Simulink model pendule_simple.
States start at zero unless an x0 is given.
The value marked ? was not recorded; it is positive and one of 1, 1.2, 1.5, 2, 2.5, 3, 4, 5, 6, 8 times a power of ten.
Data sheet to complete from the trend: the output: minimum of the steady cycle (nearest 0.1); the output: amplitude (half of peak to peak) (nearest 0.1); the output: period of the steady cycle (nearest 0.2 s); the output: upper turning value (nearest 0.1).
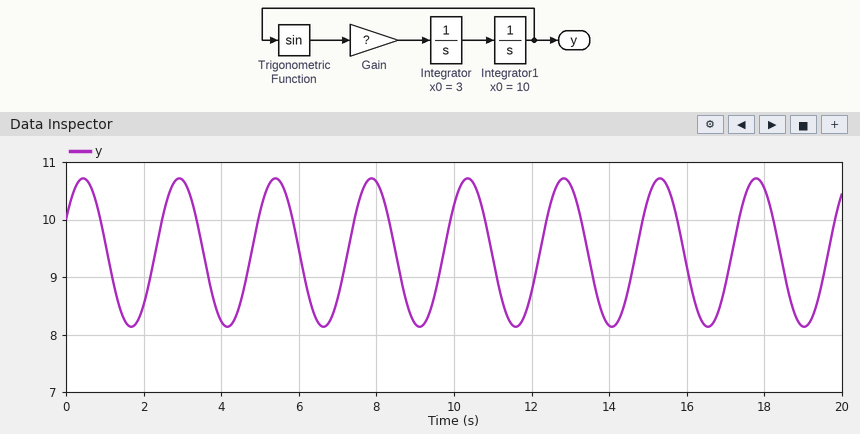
8.1
1.3
2.4 s
10.7
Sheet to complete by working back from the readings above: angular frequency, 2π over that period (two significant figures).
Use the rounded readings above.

2.6 rad/s
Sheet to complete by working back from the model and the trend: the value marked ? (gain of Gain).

8
